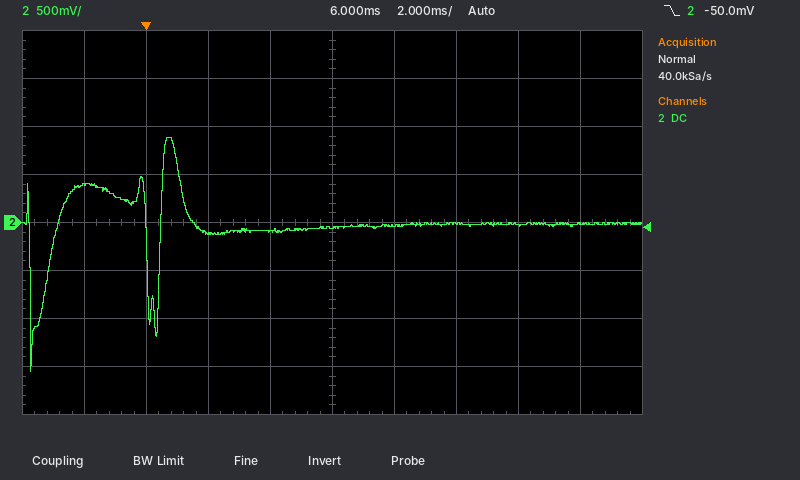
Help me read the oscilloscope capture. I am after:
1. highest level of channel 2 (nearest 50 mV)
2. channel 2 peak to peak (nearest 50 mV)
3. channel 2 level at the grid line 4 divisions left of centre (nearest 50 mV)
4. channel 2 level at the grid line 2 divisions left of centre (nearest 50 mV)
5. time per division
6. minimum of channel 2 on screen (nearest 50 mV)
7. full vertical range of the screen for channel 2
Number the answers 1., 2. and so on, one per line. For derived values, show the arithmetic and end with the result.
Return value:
1. 900 mV
2. 900 mV − (-1.55 V) = 2.45 V
3. 400 mV
4. -100 mV
5. 2 ms
6. -1.55 V
7. 4 V
